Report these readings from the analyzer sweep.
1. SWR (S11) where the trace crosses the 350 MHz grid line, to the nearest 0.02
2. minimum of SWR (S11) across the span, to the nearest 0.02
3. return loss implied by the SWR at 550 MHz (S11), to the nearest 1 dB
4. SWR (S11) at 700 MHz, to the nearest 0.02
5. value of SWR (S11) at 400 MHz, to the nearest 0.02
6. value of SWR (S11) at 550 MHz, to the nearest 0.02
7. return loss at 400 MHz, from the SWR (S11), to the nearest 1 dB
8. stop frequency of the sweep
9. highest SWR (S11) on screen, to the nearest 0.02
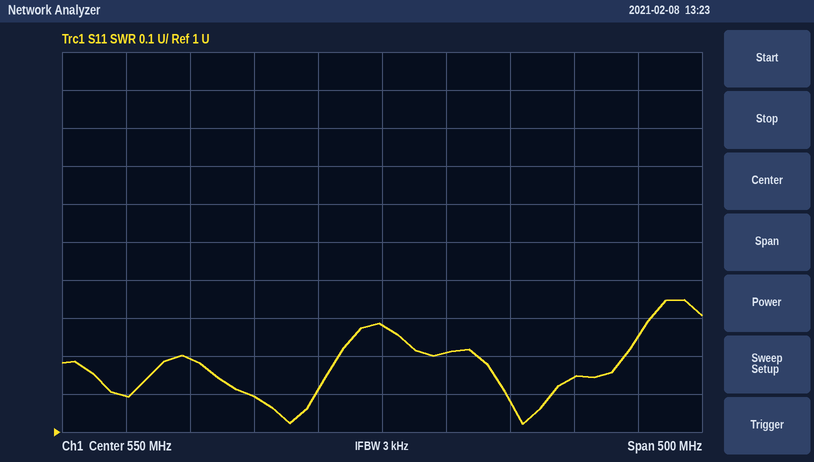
1.10
1.02
18 dB
1.14
1.20
1.28
21 dB
800 MHz
1.34
